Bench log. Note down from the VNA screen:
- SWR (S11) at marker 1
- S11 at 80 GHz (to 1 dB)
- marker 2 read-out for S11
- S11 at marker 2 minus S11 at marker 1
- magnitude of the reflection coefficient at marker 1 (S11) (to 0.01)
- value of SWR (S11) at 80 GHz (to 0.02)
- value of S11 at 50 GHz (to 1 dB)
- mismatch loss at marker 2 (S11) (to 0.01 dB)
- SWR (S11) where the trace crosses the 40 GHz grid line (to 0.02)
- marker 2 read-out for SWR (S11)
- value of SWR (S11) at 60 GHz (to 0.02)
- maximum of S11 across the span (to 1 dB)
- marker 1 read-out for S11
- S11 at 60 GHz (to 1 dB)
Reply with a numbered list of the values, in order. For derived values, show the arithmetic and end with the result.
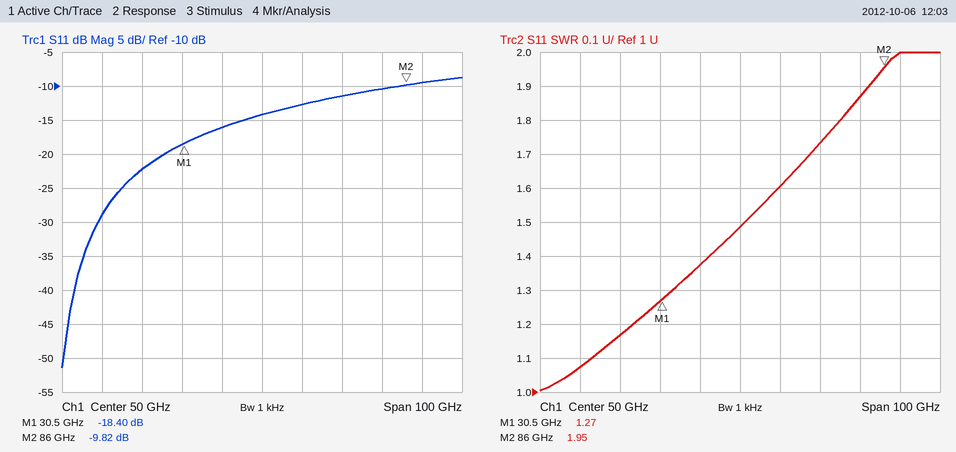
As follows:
1. 1.27
2. -10 dB
3. -9.82 dB
4. -9.82 − (-18.4) = 8.58 dB
5. 10^(-18.4/20) ≈ 0.12
6. 1.86
7. -14 dB
8. −10 log10(1 − 10^(-9.82/10)) ≈ 0.48 dB
9. 1.38
10. 1.95
11. 1.60
12. -9 dB
13. -18.40 dB
14. -13 dB
